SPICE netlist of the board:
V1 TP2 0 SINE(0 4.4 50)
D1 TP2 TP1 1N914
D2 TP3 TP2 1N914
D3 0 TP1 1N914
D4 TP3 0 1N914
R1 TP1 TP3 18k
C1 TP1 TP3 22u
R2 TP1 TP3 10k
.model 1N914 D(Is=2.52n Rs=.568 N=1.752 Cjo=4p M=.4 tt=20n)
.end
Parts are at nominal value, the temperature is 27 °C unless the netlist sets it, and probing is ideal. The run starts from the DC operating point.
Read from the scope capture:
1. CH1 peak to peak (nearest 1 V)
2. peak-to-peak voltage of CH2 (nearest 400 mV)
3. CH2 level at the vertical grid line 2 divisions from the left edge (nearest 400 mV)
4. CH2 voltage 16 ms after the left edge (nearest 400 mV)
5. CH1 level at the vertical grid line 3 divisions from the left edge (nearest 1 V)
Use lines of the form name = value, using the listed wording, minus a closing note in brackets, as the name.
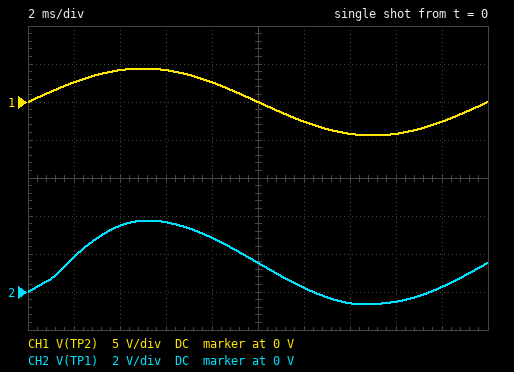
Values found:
CH1 peak to peak = 9 V
peak-to-peak voltage of CH2 = 4.4 V
CH2 level at the vertical grid line 2 divisions from the left edge = 3.6 V
CH2 voltage 16 ms after the left edge = -400 mV
CH1 level at the vertical grid line 3 divisions from the left edge = 4 V
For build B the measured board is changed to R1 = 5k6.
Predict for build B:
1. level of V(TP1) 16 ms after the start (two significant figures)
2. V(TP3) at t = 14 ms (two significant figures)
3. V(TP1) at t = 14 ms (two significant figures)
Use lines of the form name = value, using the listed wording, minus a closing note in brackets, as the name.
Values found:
level of V(TP1) 16 ms after the start = -520 mV
V(TP3) at t = 14 ms = -3.5 V
V(TP1) at t = 14 ms = -650 mV
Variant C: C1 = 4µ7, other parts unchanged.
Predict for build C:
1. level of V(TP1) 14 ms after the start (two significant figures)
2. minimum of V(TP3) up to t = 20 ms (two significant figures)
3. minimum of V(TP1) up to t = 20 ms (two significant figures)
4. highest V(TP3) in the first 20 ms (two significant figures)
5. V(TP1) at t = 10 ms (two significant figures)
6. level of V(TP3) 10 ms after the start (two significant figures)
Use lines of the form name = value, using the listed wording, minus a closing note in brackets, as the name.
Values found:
level of V(TP1) 14 ms after the start = -630 mV
minimum of V(TP3) up to t = 20 ms = -3.8 V
minimum of V(TP1) up to t = 20 ms = -640 mV
highest V(TP3) in the first 20 ms = 670 mV
V(TP1) at t = 10 ms = 1.4 V
level of V(TP3) 10 ms after the start = -1.4 V
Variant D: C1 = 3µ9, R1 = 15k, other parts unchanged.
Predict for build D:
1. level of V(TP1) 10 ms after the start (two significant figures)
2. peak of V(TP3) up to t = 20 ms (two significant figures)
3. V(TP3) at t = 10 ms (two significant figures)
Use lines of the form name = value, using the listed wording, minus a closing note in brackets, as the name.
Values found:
level of V(TP1) 10 ms after the start = 1.4 V
peak of V(TP3) up to t = 20 ms = 660 mV
V(TP3) at t = 10 ms = -1.4 V
